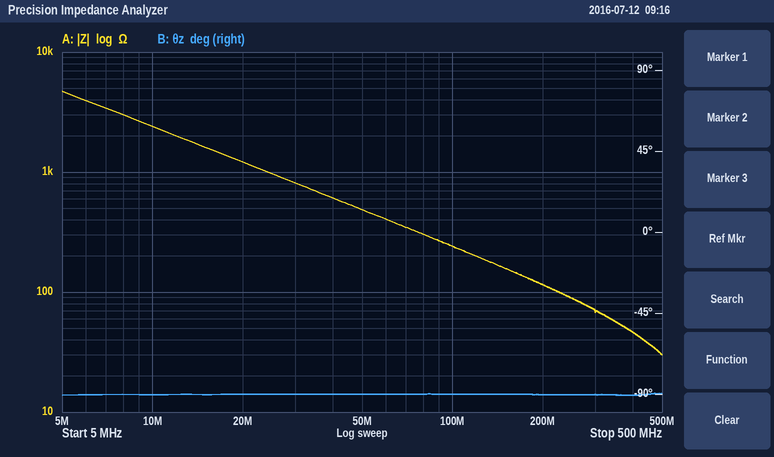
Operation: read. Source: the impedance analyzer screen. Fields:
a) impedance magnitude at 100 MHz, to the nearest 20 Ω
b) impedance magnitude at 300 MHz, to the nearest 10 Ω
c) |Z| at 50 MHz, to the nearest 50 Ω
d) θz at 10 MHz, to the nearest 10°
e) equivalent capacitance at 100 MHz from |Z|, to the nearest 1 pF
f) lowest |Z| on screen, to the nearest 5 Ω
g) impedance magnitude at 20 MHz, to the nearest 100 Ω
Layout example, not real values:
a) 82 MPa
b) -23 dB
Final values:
a) 240 Ω
b) 70 Ω
c) 500 Ω
d) -90°
e) 7 pF
f) 30 Ω
g) 1.2 kΩ
